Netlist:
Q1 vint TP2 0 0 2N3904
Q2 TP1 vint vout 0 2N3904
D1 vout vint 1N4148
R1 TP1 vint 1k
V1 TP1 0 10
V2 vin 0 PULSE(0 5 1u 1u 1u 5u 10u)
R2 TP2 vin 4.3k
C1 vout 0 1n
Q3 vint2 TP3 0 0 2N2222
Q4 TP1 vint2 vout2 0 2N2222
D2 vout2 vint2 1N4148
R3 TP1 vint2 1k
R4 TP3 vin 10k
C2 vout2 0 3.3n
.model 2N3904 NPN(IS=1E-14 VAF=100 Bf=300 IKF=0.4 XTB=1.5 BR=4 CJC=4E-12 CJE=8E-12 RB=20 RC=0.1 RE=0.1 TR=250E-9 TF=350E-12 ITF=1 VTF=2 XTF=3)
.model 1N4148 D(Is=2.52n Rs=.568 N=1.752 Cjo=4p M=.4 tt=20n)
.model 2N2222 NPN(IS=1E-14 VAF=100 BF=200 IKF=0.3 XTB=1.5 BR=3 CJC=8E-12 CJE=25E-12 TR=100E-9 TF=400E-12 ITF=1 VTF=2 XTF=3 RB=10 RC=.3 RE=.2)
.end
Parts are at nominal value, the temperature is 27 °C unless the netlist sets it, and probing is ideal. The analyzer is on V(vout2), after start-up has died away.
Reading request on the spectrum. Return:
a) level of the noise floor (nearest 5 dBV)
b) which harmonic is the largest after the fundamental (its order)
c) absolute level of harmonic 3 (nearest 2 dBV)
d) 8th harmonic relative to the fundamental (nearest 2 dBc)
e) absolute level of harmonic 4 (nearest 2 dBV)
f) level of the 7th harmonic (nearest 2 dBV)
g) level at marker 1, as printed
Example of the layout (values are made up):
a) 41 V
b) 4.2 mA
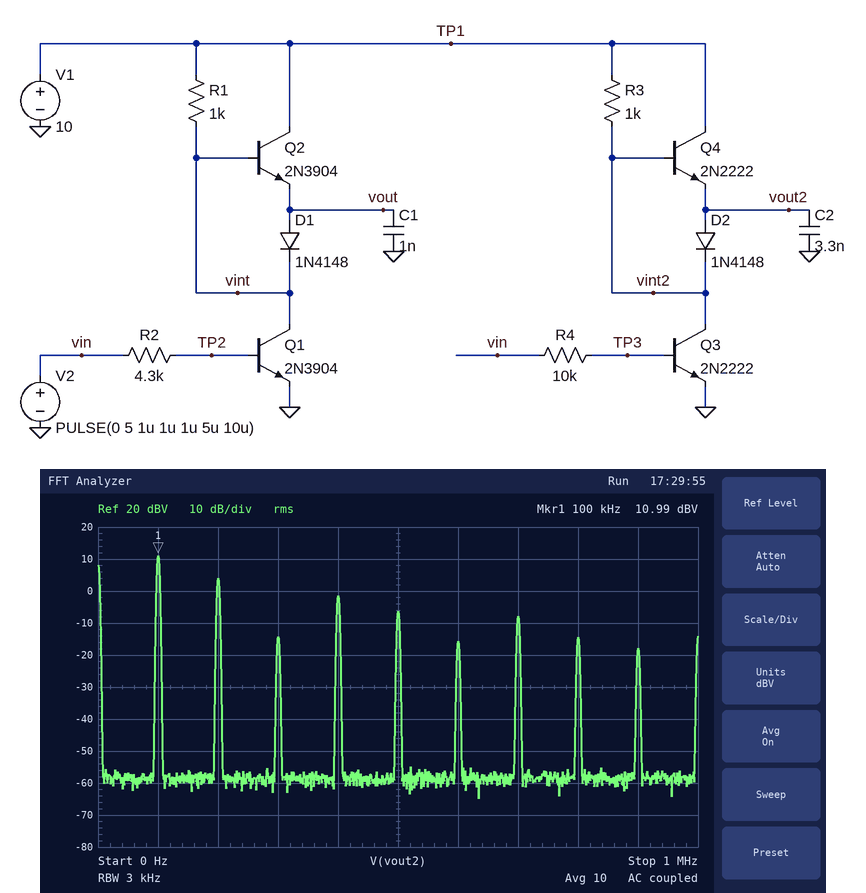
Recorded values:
a) -60 dBV
b) 2
c) -14 dBV
d) -26 dBc
e) -2 dBV
f) -8 dBV
g) 10.99 dBV
